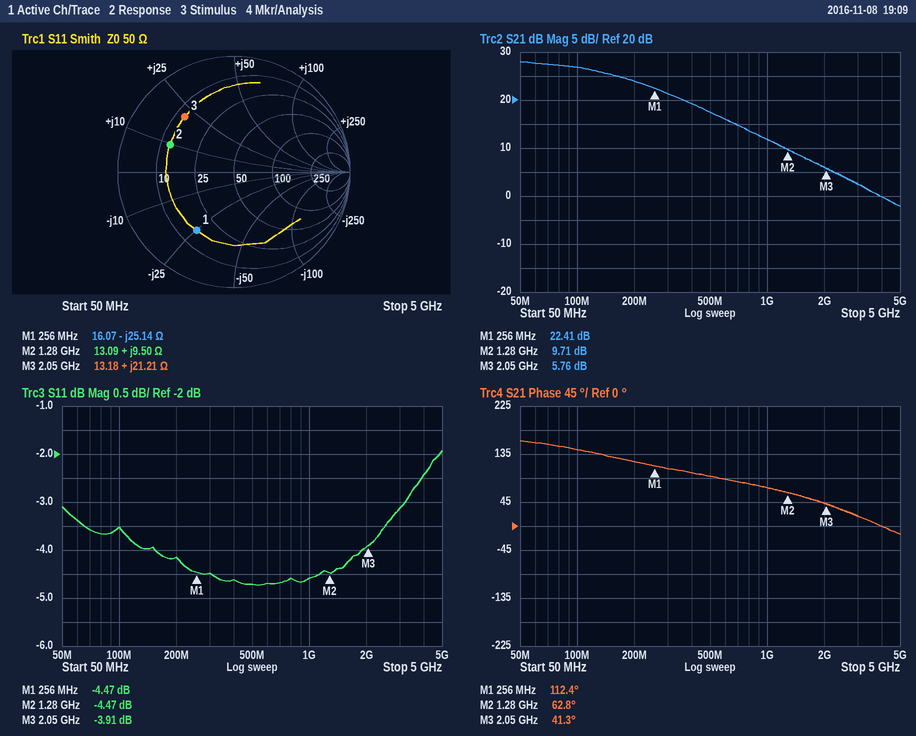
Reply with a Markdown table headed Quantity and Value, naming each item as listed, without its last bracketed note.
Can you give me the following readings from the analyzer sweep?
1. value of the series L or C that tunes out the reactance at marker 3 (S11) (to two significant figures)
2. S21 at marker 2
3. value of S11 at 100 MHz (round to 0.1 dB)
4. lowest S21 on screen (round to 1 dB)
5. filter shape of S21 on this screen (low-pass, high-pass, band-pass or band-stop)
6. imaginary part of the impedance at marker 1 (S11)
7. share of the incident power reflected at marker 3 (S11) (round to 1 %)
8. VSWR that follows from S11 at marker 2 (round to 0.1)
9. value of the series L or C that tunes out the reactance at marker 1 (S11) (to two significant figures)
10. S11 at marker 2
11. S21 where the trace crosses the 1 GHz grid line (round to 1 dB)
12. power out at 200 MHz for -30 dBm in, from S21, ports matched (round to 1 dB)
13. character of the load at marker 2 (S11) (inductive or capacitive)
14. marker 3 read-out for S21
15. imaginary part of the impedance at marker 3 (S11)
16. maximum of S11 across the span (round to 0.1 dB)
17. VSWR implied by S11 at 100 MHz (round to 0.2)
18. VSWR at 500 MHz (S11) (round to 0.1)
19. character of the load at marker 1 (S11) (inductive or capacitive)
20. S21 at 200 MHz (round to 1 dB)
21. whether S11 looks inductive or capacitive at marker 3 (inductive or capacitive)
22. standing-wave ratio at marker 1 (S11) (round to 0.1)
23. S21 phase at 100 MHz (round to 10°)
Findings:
| Quantity | Value |
|---|---|
| value of the series L or C that tunes out the reactance at marker 3 (S11) | 3.7 pF |
| S21 at marker 2 | 9.71 dB |
| value of S11 at 100 MHz | -3.5 dB |
| lowest S21 on screen | -2 dB |
| filter shape of S21 on this screen | low-pass |
| imaginary part of the impedance at marker 1 | -25.14 Ω |
| share of the incident power reflected at marker 3 (S11) | 41 % |
| VSWR that follows from S11 at marker 2 | 4.0 |
| value of the series L or C that tunes out the reactance at marker 1 (S11) | 16 nH |
| S11 at marker 2 | -4.47 dB |
| S21 where the trace crosses the 1 GHz grid line | 12 dB |
| power out at 200 MHz for -30 dBm in, from S21, ports matched | -6 dBm |
| character of the load at marker 2 (S11) | inductive |
| marker 3 read-out for S21 | 5.76 dB |
| imaginary part of the impedance at marker 3 | +21.21 Ω |
| maximum of S11 across the span | -1.9 dB |
| VSWR implied by S11 at 100 MHz | 5.0 |
| VSWR at 500 MHz (S11) | 3.8 |
| character of the load at marker 1 (S11) | capacitive |
| S21 at 200 MHz | 24 dB |
| whether S11 looks inductive or capacitive at marker 3 | inductive |
| standing-wave ratio at marker 1 (S11) | 4.0 |
| S21 phase at 100 MHz | 140° |
